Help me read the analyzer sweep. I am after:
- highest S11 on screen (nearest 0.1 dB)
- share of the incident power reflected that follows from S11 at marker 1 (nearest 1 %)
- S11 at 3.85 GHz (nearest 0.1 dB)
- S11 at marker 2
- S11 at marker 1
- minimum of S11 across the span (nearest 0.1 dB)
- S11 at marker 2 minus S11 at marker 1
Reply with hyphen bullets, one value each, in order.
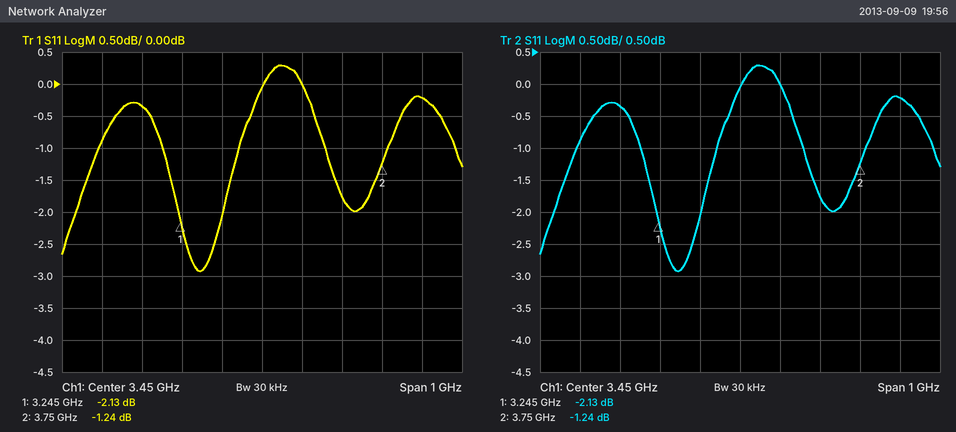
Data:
- 0.3 dB
- 61 %
- -0.2 dB
- -1.24 dB
- -2.13 dB
- -2.9 dB
- 0.89 dB
